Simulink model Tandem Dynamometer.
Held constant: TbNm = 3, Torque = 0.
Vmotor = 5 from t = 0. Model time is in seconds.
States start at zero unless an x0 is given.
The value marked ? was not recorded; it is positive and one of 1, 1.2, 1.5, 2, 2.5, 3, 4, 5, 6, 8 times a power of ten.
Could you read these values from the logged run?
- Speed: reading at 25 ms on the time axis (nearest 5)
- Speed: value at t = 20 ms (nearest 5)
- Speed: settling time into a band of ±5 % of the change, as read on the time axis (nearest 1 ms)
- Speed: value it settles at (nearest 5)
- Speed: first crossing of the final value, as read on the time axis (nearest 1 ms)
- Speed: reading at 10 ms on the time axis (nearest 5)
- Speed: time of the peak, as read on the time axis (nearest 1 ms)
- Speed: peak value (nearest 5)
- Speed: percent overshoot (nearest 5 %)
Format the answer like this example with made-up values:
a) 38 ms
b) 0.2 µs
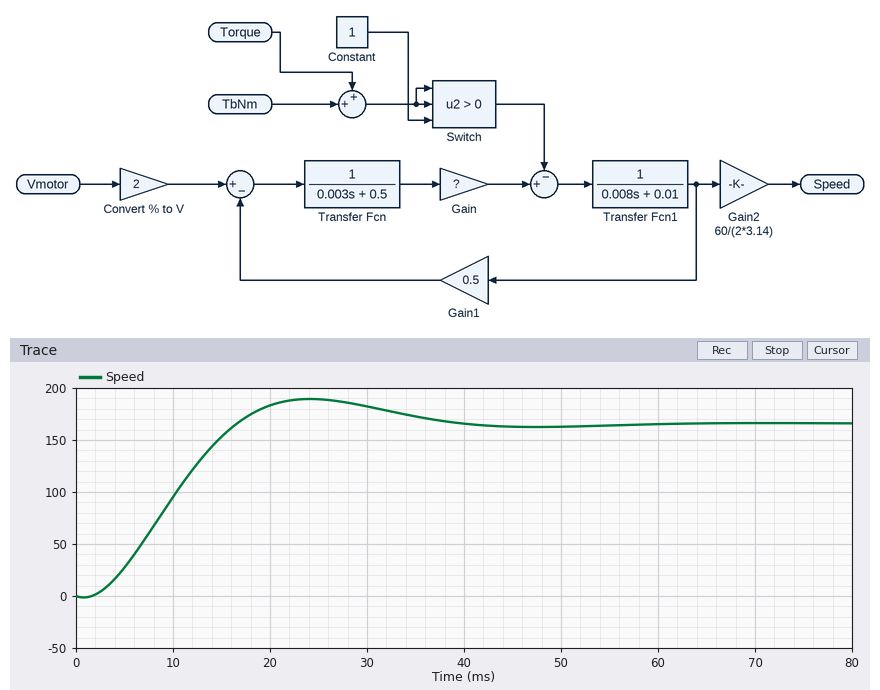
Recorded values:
a) 190
b) 185
c) 34 ms
d) 165
e) 17 ms
f) 95
g) 24 ms
h) 190
i) 15 %
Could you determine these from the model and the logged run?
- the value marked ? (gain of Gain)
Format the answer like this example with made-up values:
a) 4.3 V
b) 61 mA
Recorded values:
a) 1.2
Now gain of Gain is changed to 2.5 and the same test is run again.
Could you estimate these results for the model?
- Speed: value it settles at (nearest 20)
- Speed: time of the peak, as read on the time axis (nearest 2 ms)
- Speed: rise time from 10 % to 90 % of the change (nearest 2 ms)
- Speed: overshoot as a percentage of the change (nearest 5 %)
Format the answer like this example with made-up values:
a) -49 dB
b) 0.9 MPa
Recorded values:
a) 180
b) 16 ms
c) 6 ms
d) 30 %
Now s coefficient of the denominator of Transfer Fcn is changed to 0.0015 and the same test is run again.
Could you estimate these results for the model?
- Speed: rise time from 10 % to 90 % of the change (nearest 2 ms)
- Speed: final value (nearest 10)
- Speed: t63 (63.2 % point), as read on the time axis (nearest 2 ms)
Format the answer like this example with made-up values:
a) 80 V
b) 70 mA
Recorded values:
a) 10 ms
b) 170
c) 8 ms
